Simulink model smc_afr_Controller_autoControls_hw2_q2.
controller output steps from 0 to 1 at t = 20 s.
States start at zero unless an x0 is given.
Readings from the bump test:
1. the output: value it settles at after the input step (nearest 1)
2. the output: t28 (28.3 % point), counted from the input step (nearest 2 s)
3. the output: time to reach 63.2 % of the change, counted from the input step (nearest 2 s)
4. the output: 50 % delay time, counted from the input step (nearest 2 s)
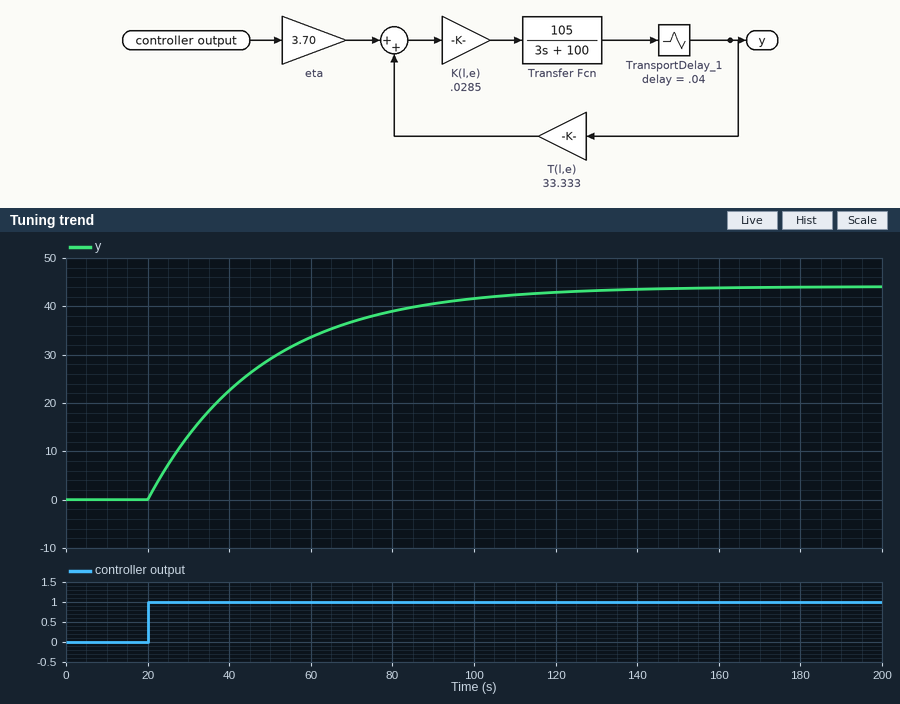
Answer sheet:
44
10 s
28 s
20 s
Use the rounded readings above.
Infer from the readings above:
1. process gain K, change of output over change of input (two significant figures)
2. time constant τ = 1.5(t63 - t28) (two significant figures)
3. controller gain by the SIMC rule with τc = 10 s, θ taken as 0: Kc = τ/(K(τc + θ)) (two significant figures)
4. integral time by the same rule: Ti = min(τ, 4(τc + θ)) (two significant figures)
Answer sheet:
44
27 s
0.061
27 s
